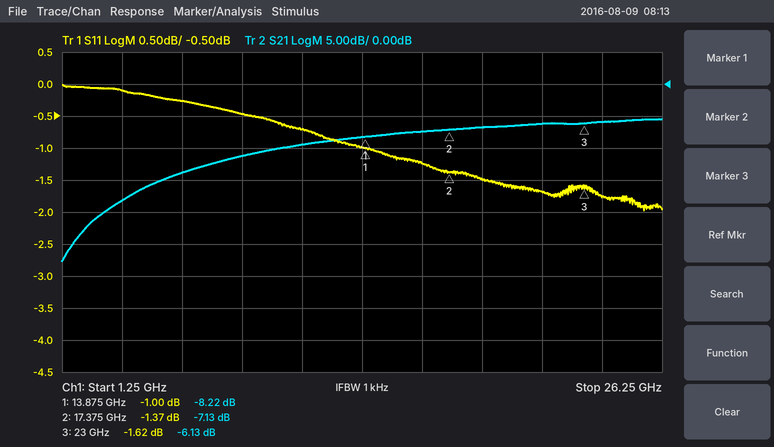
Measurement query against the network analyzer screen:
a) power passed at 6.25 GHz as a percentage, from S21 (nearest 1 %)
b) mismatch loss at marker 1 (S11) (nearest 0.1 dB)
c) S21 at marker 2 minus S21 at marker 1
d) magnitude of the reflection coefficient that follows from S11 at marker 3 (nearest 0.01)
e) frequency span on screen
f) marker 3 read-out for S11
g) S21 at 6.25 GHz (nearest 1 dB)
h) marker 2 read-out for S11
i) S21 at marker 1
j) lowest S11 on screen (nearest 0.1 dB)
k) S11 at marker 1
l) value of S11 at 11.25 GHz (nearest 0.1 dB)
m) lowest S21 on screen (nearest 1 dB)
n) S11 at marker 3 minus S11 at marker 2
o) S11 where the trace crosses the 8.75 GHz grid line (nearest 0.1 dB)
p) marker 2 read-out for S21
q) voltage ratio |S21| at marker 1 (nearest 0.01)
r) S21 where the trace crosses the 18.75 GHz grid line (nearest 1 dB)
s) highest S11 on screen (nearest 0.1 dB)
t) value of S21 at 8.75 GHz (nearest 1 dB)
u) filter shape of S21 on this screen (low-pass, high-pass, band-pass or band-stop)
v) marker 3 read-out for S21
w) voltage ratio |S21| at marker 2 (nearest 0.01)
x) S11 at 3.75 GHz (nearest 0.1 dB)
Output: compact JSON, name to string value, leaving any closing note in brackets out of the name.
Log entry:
{"power passed at 6.25 GHz as a percentage, from S21": "4 %", "mismatch loss at marker 1 (S11)": "6.9 dB", "S21 at marker 2 minus S21 at marker 1": "1.09 dB", "magnitude of the reflection coefficient that follows from S11 at marker 3": "0.83", "frequency span on screen": "25 GHz", "marker 3 read-out for S11": "-1.62 dB", "S21 at 6.25 GHz": "-14 dB", "marker 2 read-out for S11": "-1.37 dB", "S21 at marker 1": "-8.22 dB", "lowest S11 on screen": "-2.0 dB", "S11 at marker 1": "-1.00 dB", "value of S11 at 11.25 GHz": "-0.7 dB", "lowest S21 on screen": "-28 dB", "S11 at marker 3 minus S11 at marker 2": "-0.25 dB", "S11 where the trace crosses the 8.75 GHz grid line": "-0.5 dB", "marker 2 read-out for S21": "-7.13 dB", "voltage ratio |S21| at marker 1": "0.39", "S21 where the trace crosses the 18.75 GHz grid line": "-7 dB", "highest S11 on screen": "0.0 dB", "value of S21 at 8.75 GHz": "-11 dB", "filter shape of S21 on this screen": "high-pass", "marker 3 read-out for S21": "-6.13 dB", "voltage ratio |S21| at marker 2": "0.44", "S11 at 3.75 GHz": "-0.1 dB"}
